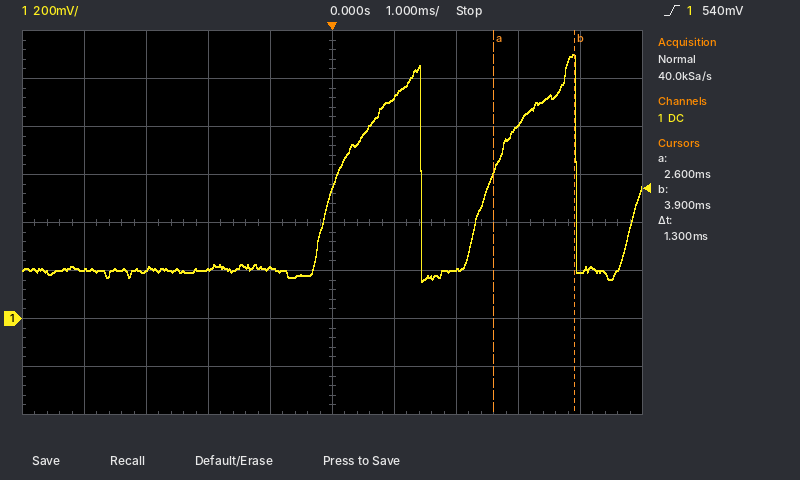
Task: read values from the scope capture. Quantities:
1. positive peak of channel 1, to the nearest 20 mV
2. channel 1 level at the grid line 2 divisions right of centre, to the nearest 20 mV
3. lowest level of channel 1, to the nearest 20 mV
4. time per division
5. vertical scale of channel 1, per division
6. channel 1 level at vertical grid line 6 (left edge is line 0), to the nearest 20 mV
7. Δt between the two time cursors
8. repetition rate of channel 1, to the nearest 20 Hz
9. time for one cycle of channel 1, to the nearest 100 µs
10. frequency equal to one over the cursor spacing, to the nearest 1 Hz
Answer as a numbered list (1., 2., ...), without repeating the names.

1. 1.10 V
2. 200 mV
3. 160 mV
4. 1 ms
5. 200 mV
6. 920 mV
7. 1.3 ms
8. 400 Hz
9. 2.5 ms
10. 769 Hz
